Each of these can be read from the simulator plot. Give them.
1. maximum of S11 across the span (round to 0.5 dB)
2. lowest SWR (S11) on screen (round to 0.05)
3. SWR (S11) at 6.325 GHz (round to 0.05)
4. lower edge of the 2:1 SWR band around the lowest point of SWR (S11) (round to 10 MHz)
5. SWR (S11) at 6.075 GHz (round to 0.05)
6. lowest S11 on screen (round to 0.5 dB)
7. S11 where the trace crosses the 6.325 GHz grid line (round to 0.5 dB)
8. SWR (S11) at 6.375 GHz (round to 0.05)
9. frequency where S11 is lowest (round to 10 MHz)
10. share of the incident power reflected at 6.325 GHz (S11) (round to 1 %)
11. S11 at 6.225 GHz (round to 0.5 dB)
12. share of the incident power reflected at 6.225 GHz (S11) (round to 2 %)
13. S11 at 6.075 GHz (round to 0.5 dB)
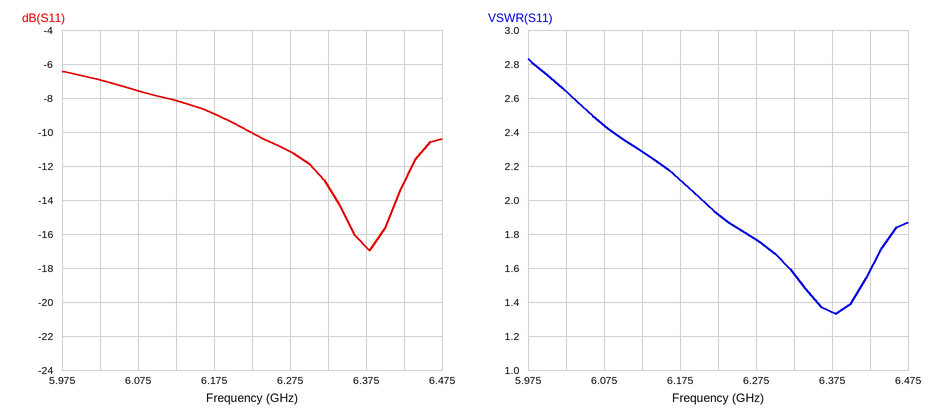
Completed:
-6.5 dB
1.35
1.55
6.20 GHz
2.45
-17.0 dB
-13.0 dB
1.35
6.38 GHz
5 %
-10.0 dB
10 %
-7.5 dB
